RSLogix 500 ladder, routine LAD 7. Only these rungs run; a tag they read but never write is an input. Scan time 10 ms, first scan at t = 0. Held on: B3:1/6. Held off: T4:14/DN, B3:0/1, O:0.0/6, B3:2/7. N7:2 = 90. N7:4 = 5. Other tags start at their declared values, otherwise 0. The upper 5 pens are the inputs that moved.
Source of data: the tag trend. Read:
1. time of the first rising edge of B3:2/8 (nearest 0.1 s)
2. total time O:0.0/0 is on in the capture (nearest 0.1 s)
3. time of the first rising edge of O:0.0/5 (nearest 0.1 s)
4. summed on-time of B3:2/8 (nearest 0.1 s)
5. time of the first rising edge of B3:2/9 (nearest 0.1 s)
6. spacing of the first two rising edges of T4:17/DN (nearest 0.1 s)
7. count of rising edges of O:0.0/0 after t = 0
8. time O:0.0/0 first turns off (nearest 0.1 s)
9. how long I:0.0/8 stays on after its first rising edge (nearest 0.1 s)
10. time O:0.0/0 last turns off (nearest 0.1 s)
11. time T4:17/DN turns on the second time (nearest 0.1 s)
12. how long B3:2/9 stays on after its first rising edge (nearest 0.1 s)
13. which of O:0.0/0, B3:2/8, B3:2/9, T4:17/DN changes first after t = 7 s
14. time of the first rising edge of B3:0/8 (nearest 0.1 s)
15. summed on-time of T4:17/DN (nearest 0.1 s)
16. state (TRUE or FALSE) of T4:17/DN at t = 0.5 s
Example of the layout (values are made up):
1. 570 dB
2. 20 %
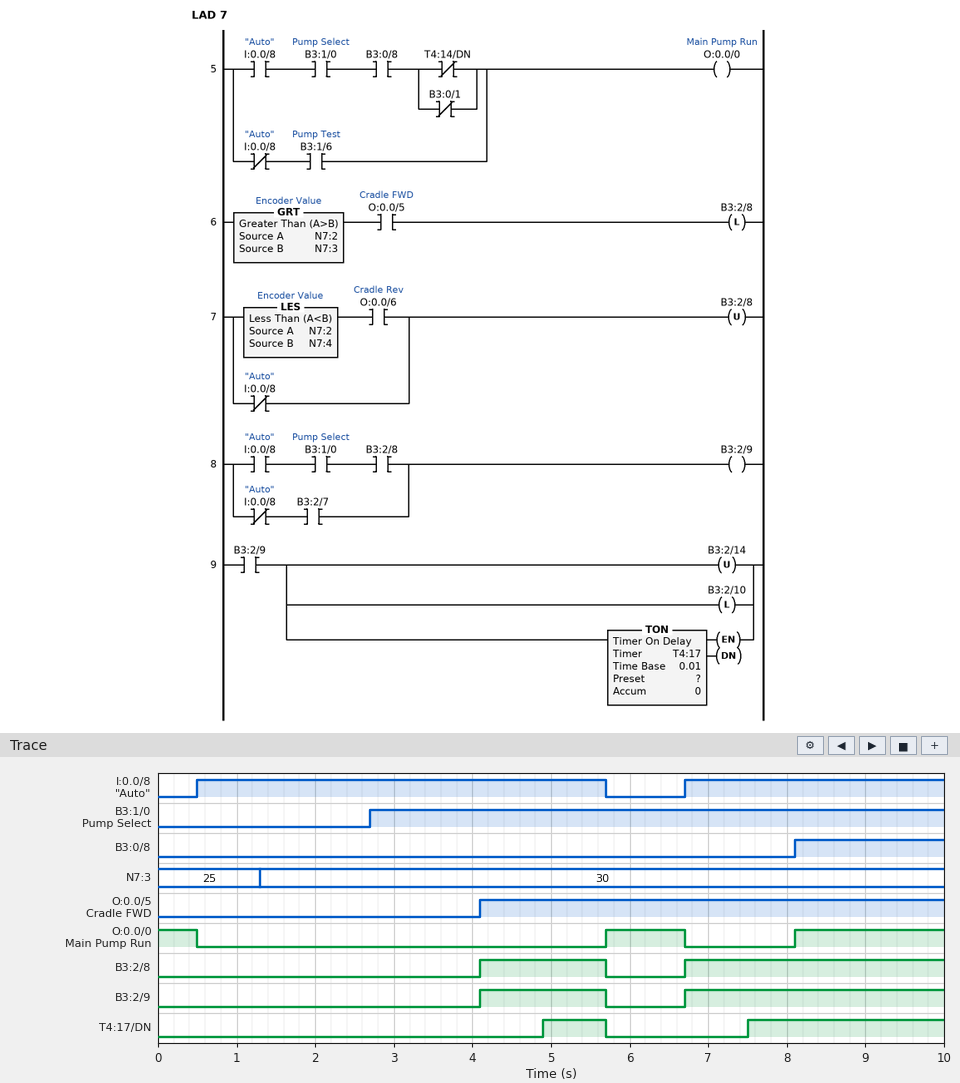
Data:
1. 4.1 s
2. 3.4 s
3. 4.1 s
4. 4.9 s
5. 4.1 s
6. 2.6 s
7. 2
8. 0.5 s
9. 5.2 s
10. 6.7 s
11. 7.5 s
12. 1.6 s
13. T4:17/DN
14. 8.1 s
15. 3.3 s
16. FALSE
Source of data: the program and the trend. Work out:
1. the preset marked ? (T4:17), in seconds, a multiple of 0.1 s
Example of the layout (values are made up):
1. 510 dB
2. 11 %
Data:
1. 0.8 s
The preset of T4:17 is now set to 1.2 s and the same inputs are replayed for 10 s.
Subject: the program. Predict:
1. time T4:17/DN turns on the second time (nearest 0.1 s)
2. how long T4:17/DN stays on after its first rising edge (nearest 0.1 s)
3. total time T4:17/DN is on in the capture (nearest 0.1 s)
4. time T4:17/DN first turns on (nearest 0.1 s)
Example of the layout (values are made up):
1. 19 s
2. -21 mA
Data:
1. 7.9 s
2. 0.4 s
3. 2.5 s
4. 5.3 s
